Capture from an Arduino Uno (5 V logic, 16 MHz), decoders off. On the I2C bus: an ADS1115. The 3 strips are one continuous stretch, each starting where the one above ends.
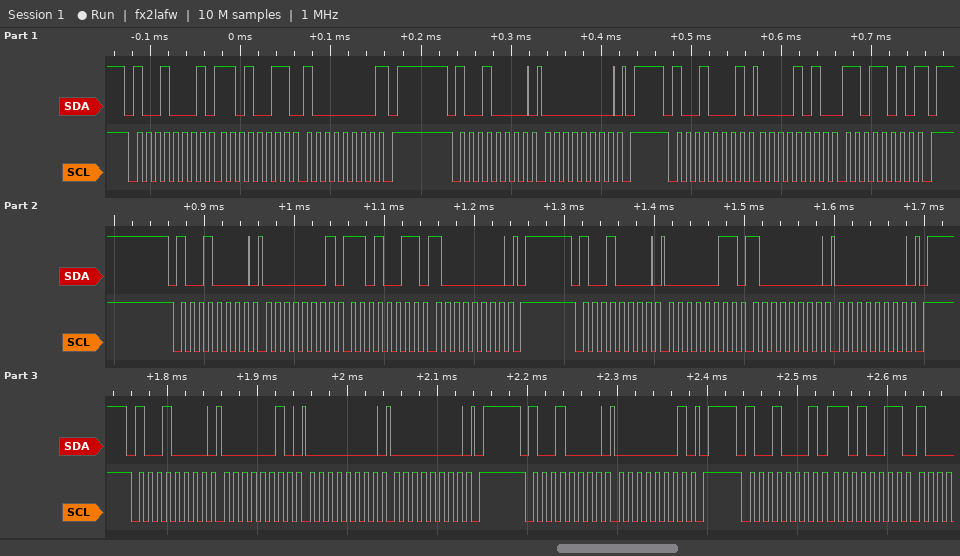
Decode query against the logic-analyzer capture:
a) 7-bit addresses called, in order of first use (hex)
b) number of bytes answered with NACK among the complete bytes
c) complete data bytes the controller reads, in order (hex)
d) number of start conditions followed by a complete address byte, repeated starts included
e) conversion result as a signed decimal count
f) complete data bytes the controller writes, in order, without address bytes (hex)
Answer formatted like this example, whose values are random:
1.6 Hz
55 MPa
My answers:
0x48
2
D3 80 0A DA D3
8
2778
00 01 D3 80 03 80 00 02 00 00 01
